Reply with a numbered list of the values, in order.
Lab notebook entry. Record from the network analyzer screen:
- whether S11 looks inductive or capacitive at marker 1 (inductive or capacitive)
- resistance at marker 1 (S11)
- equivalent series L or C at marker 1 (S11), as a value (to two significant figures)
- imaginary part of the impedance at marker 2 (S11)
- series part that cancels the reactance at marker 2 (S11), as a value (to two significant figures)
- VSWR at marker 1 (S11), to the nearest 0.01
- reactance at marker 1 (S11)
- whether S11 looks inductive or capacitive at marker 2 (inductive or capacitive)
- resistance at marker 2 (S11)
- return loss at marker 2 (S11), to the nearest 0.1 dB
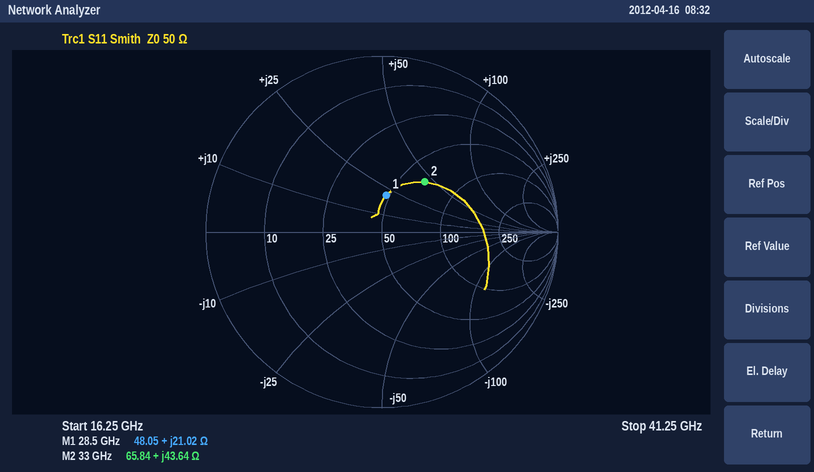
1. inductive
2. 48.05 Ω
3. 120 pH
4. +43.64 Ω
5. 110 fF
6. 1.53
7. +21.02 Ω
8. inductive
9. 65.84 Ω
10. 8.5 dB
